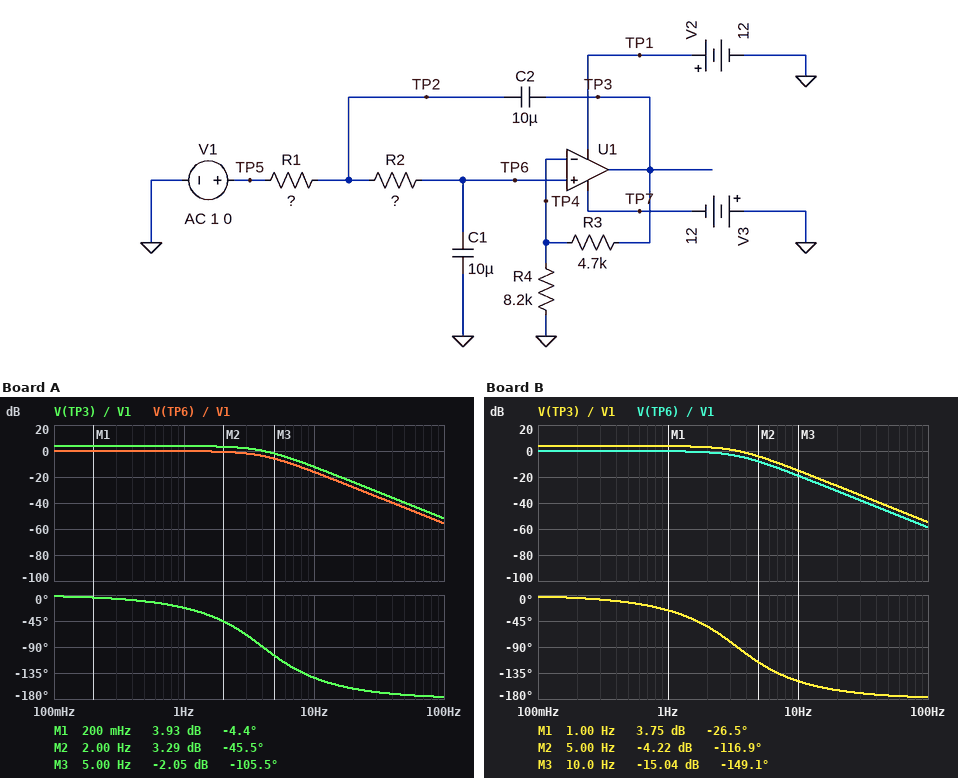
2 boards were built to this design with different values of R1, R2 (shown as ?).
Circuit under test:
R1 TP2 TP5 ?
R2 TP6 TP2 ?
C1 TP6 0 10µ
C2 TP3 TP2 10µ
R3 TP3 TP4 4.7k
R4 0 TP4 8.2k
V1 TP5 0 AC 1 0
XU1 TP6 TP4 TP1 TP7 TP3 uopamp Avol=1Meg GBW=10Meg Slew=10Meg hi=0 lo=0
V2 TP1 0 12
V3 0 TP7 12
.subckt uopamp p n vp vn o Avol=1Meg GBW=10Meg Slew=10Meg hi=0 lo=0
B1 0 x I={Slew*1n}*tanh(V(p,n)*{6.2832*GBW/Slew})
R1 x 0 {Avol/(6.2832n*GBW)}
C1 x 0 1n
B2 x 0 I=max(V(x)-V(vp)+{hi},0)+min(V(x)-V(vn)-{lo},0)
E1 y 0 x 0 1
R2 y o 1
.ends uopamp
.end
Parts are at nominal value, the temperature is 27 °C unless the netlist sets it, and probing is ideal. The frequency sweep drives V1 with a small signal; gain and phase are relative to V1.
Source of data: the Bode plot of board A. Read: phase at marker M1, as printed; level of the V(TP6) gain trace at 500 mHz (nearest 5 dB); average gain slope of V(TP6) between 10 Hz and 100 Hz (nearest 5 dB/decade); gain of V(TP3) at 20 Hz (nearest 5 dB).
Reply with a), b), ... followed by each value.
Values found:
a) -4.4 deg
b) 0 dB
c) -40 dB/decade
d) -25 dB
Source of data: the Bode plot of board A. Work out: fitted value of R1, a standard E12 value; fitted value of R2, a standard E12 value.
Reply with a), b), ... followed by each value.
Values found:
a) 3.3 kΩ
b) 4.7 kΩ
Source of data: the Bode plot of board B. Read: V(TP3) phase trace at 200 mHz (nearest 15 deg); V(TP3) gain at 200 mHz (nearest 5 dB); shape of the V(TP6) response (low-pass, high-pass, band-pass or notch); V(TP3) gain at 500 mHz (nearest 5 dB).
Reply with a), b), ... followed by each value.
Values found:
a) 0 deg
b) 5 dB
c) low-pass
d) 5 dB
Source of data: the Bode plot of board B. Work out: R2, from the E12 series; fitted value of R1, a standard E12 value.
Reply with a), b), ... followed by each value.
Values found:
a) 5.6 kΩ
b) 3.9 kΩ
